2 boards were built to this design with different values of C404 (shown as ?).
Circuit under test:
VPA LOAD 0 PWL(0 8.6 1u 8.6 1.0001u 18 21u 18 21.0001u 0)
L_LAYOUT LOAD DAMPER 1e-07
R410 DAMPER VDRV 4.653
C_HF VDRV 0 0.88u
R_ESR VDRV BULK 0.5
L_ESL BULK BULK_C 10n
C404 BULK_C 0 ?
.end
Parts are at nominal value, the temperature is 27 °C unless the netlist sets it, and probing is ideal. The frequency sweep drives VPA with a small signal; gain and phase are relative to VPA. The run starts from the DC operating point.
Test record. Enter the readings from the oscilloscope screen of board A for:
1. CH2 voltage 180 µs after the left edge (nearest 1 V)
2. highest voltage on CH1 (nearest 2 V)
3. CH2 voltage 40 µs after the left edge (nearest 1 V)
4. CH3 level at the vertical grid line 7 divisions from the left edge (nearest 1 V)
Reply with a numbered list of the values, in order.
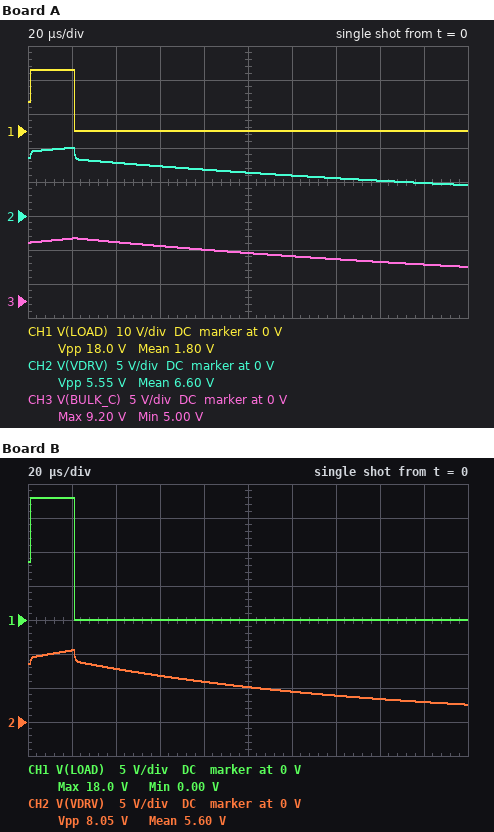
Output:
1. 5 V
2. 18 V
3. 8 V
4. 6 V
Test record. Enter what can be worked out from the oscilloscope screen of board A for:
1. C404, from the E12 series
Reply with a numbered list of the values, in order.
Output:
1. 56 µF
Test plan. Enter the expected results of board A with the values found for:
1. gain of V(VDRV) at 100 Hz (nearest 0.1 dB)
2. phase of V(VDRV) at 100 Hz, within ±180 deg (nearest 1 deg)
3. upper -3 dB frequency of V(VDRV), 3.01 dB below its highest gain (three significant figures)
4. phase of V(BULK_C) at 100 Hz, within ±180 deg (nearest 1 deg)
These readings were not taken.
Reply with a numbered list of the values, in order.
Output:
1. -0.1 dB
2. -9 deg
3. 550 Hz
4. -10 deg
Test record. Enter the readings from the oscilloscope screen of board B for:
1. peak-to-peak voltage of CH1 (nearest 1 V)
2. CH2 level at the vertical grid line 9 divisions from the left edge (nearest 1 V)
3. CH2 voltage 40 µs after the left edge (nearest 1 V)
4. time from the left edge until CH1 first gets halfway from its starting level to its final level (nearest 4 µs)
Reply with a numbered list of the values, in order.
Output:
1. 18 V
2. 3 V
3. 8 V
4. 20 µs
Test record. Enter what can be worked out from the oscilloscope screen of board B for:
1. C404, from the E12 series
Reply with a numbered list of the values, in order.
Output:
1. 27 µF
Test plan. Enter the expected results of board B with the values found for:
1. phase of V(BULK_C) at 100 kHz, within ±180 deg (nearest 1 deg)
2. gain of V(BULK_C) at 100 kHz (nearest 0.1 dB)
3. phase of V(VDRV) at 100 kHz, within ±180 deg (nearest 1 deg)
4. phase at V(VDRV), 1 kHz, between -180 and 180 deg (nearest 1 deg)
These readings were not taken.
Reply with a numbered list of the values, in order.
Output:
1. -104 deg
2. -39.3 dB
3. -20 deg
4. -37 deg
